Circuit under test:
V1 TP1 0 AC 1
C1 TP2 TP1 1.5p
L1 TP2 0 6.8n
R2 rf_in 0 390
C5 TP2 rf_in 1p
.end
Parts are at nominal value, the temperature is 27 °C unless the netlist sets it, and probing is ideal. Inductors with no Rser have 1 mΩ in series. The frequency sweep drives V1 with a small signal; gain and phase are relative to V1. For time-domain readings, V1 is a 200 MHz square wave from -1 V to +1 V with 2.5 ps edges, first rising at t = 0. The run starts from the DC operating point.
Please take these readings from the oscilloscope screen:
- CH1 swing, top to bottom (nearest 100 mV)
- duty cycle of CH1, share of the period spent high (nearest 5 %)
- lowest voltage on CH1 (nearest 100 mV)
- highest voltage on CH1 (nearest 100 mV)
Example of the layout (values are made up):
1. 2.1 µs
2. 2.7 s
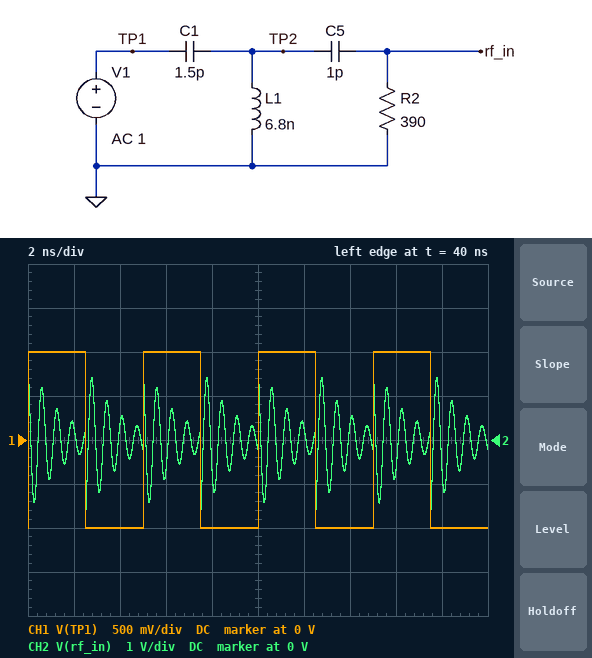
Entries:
1. 2.0 V
2. 50 %
3. -1.0 V
4. 1.0 V
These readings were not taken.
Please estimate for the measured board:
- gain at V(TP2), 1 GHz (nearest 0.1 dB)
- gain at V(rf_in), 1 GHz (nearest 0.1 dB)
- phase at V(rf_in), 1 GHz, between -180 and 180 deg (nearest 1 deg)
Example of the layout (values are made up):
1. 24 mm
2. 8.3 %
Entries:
1. -3.0 dB
2. -3.6 dB
3. -167 deg
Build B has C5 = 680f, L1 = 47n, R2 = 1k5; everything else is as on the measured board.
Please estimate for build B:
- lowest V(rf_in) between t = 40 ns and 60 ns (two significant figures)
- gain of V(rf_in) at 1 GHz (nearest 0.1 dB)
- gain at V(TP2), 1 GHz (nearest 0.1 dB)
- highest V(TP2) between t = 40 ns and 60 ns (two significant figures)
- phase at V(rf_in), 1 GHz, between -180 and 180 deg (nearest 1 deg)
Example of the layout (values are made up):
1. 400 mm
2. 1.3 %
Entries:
1. -4.7 V
2. 3.6 dB
3. 3.7 dB
4. 4.7 V
5. 15 deg
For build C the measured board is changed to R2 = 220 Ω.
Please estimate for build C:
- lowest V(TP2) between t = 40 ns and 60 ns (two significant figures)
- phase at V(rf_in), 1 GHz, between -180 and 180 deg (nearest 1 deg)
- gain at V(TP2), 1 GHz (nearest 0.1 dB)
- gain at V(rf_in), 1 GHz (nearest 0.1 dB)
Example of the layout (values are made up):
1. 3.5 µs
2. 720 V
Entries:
1. -2.0 V
2. -158 deg
3. -2.2 dB
4. -4.1 dB
